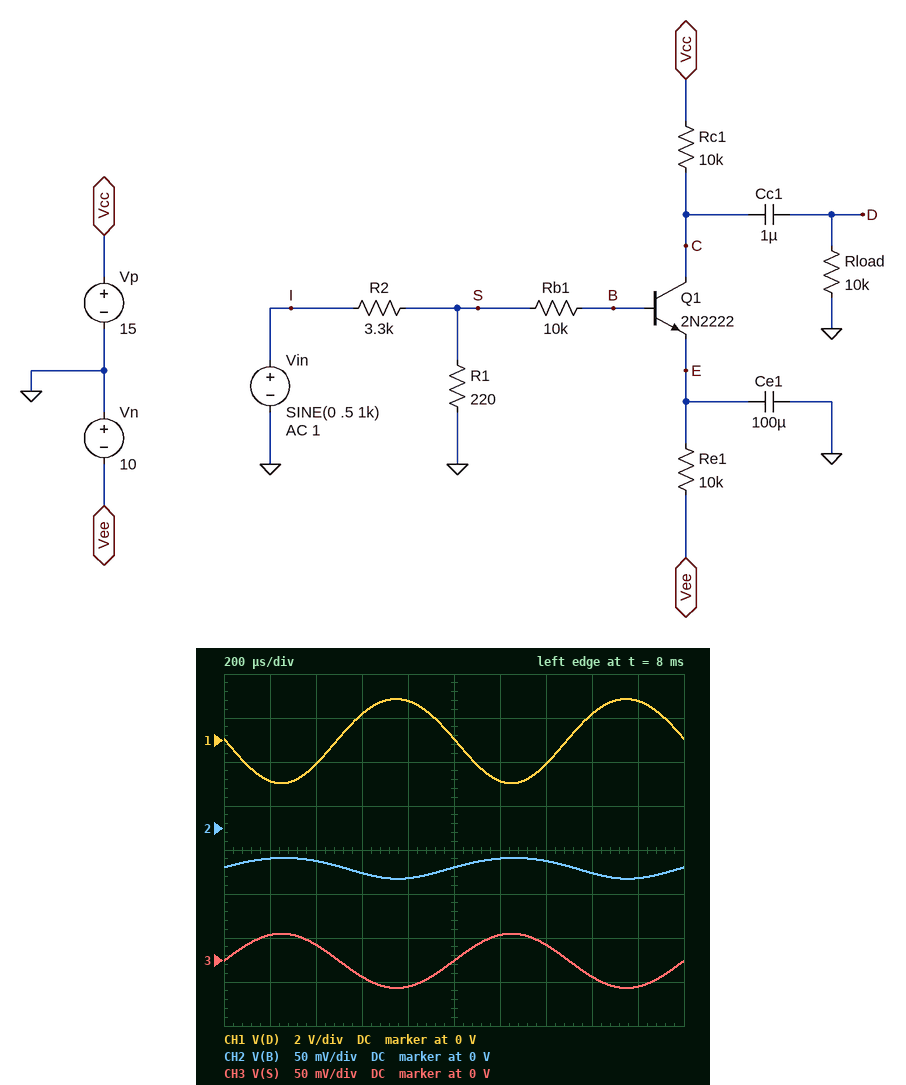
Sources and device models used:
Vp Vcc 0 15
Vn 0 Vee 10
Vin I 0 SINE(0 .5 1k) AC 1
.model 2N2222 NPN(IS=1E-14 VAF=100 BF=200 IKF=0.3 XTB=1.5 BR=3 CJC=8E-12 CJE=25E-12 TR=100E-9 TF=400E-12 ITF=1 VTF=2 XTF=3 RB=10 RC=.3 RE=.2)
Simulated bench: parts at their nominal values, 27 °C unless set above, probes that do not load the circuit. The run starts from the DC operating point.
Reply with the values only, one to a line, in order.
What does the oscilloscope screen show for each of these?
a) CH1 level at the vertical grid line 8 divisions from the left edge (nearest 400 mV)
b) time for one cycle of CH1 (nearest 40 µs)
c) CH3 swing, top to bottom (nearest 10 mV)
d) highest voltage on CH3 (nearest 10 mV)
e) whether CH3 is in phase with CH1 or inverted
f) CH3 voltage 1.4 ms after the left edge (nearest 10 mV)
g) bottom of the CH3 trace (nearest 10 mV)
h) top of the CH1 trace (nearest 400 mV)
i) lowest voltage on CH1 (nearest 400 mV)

1.2 V
1.00 ms
60 mV
30 mV
inverted
20 mV
-30 mV
2.0 V
-2.0 V
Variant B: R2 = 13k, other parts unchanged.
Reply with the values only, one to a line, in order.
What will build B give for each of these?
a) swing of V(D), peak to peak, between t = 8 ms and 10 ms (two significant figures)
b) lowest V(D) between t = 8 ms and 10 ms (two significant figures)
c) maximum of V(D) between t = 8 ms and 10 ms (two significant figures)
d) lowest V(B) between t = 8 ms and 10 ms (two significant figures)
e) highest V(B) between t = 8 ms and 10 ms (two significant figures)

1.0 V
-520 mV
520 mV
-48 mV
-42 mV
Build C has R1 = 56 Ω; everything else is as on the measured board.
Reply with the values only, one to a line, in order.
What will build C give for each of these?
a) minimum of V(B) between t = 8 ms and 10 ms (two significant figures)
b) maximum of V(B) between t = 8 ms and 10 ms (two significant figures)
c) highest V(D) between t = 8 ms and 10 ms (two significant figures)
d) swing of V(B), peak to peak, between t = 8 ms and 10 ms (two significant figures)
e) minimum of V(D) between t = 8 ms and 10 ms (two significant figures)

-47 mV
-41 mV
520 mV
6.2 mV
-530 mV
